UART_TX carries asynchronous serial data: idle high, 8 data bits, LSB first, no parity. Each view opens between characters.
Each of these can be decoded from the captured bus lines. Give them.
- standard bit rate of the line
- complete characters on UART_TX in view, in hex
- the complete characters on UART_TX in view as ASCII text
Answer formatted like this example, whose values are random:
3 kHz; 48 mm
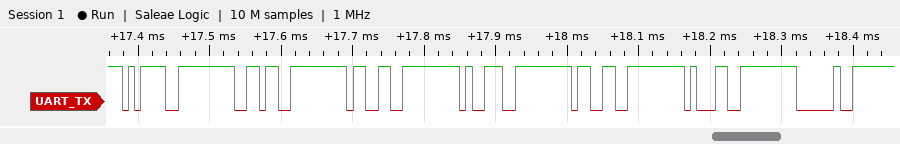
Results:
115200 baud; 3D, 36, 33, 39, 33, 31, 20; "=63931 "
